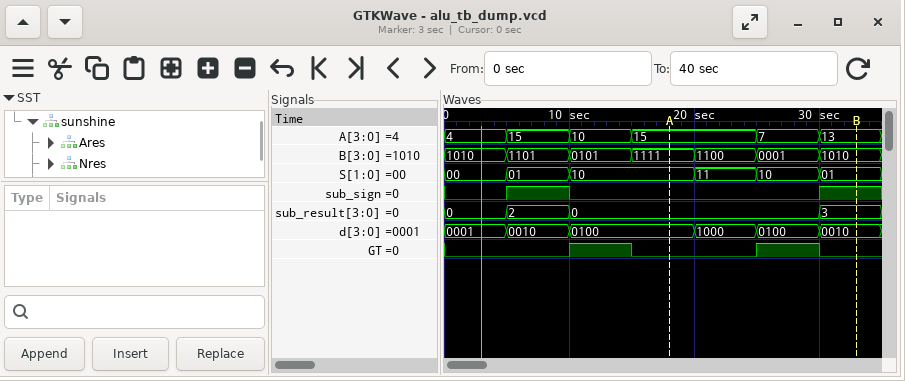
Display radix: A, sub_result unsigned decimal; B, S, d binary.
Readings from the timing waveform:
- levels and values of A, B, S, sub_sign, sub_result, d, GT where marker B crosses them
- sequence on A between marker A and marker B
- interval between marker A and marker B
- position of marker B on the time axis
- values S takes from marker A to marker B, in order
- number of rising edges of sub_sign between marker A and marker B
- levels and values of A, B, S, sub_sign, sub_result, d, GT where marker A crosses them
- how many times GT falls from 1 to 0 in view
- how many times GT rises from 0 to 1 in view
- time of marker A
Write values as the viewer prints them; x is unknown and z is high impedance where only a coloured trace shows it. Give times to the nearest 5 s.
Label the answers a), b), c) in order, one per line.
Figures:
a) A=13, B=1010, S=01, sub_sign=1, sub_result=3, d=0010, GT=0
b) 15, 7, 13
c) 15 s
d) 35 s
e) 10, 11, 10, 01
f) 1
g) A=15, B=1111, S=10, sub_sign=0, sub_result=0, d=0100, GT=0
h) 2
i) 2
j) 20 s
